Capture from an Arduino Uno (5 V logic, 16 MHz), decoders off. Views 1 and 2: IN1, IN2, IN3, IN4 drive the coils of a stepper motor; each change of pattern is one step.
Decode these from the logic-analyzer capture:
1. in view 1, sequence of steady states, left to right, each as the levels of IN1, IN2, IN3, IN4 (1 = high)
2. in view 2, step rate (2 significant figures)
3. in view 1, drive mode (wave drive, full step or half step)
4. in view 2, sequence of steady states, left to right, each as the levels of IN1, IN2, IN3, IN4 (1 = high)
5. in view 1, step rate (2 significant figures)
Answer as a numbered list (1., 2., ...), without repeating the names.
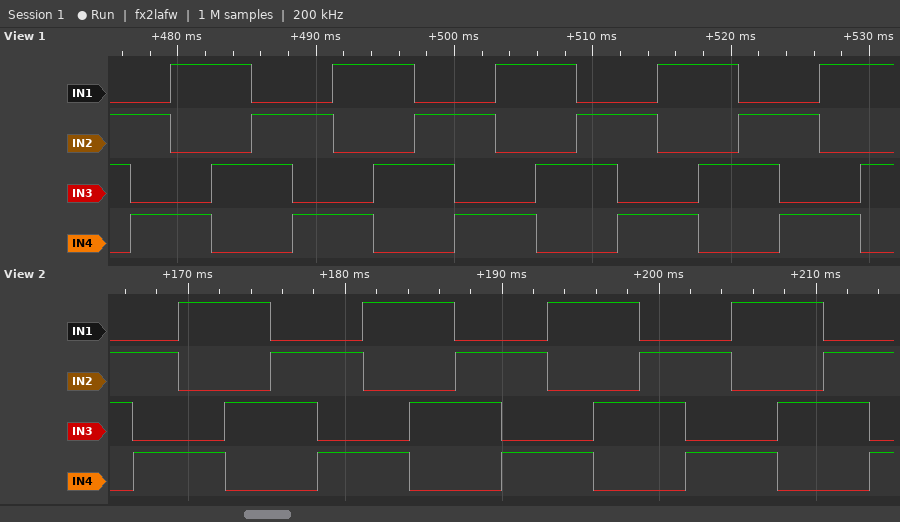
1. 0110 0101 1001 1010 0110 0101 1001 1010 0110 0101 1001 1010 0110 0101 1001 1010 0110 0101 1001 1010
2. 340 steps/s
3. full step
4. 0110 0101 1001 1010 0110 0101 1001 1010 0110 0101 1001 1010 0110 0101 1001 1010 0110 0101
5. 340 steps/s
